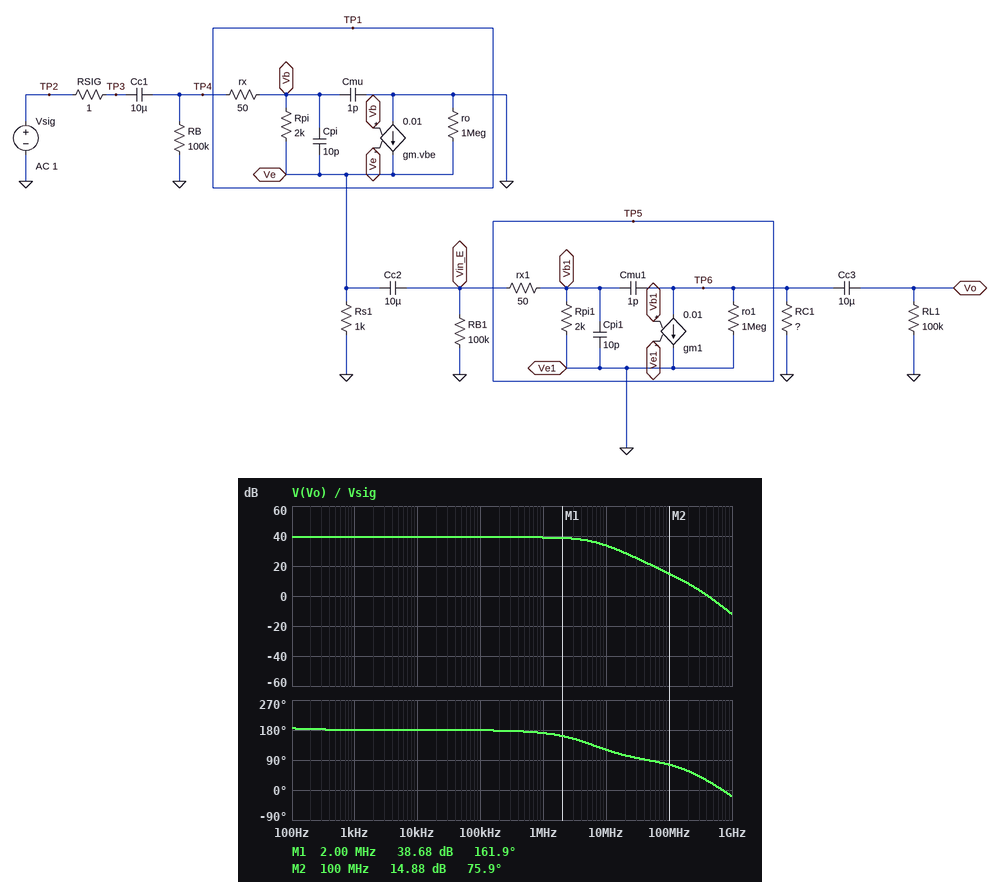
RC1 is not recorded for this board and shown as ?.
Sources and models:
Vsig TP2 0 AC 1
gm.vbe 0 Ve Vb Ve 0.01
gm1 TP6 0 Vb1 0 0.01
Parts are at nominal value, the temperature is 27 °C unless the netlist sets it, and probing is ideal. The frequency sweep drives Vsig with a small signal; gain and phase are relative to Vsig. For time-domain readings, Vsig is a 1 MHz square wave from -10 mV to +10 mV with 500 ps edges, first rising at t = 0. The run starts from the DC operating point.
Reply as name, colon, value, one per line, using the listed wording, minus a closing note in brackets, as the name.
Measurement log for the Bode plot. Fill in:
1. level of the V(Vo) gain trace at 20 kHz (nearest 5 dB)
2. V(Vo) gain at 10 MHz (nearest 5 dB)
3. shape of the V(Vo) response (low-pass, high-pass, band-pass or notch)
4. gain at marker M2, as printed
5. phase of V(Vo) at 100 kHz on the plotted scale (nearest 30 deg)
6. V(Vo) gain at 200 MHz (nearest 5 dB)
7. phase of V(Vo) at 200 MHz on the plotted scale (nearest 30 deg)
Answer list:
level of the V(Vo) gain trace at 20 kHz: 40 dB
V(Vo) gain at 10 MHz: 35 dB
shape of the V(Vo) response: low-pass
gain at marker M2, as printed: 14.88 dB
phase of V(Vo) at 100 kHz on the plotted scale: 180 deg
V(Vo) gain at 200 MHz: 10 dB
phase of V(Vo) at 200 MHz on the plotted scale: 60 deg
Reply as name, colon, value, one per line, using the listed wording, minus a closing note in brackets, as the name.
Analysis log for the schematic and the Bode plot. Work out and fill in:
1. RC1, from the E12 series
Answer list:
RC1, from the E12 series: 12 kΩ
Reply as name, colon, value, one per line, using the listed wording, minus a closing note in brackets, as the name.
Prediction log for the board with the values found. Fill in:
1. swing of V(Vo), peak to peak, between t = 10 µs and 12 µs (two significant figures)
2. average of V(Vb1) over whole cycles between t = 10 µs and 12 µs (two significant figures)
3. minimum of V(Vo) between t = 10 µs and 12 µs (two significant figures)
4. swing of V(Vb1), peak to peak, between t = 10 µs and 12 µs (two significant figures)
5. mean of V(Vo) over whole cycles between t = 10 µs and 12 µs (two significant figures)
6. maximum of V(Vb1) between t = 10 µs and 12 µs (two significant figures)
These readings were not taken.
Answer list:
swing of V(Vo), peak to peak, between t = 10 µs and 12 µs: 1.8 V
average of V(Vb1) over whole cycles between t = 10 µs and 12 µs: 8.5 mV
minimum of V(Vo) between t = 10 µs and 12 µs: -1.8 V
swing of V(Vb1), peak to peak, between t = 10 µs and 12 µs: 17 mV
mean of V(Vo) over whole cycles between t = 10 µs and 12 µs: -900 mV
maximum of V(Vb1) between t = 10 µs and 12 µs: 17 mV
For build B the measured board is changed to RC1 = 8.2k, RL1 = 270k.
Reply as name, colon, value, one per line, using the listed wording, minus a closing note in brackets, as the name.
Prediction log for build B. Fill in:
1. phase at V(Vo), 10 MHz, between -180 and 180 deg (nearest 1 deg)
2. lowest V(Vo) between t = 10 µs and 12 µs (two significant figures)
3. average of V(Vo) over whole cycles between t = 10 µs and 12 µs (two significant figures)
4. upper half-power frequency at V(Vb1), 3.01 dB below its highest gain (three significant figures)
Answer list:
phase at V(Vo), 10 MHz, between -180 and 180 deg: 128 deg
lowest V(Vo) between t = 10 µs and 12 µs: -1.3 V
average of V(Vo) over whole cycles between t = 10 µs and 12 µs: -670 mV
upper half-power frequency at V(Vb1), 3.01 dB below its highest gain: 10.2 MHz
